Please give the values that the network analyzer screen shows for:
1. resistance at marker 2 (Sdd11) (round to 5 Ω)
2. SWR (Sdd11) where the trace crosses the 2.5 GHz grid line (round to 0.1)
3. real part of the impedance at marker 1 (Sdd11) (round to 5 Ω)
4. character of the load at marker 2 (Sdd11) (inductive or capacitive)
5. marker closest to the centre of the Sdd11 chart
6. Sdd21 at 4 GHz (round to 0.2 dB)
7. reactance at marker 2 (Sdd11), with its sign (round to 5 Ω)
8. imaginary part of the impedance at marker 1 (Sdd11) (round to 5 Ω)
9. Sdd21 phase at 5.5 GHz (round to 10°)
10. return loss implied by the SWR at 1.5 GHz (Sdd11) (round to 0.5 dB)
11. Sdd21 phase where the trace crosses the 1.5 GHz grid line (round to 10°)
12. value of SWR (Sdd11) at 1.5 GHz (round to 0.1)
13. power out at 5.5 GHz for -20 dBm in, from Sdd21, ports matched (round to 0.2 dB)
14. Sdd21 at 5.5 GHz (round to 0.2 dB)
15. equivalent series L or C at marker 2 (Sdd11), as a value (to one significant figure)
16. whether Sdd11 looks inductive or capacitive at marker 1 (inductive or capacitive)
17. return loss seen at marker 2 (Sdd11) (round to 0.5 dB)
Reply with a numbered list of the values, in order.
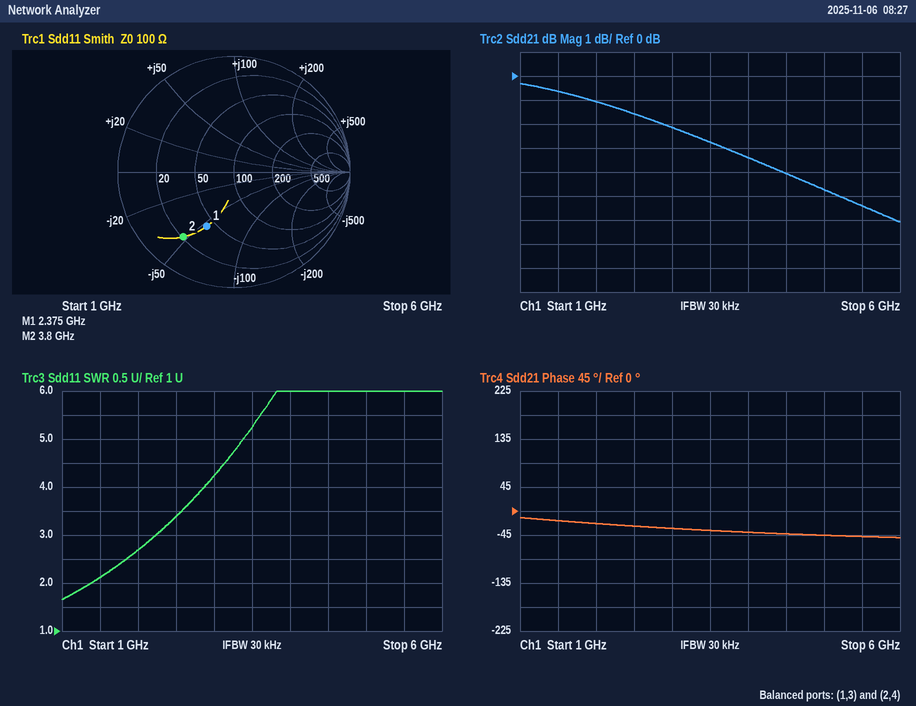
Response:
1. 20 Ω
2. 3.4
3. 40 Ω
4. capacitive
5. marker 1
6. -3.4 dB
7. -45 Ω
8. -55 Ω
9. -50°
10. 9.0 dB
11. -20°
12. 2.1
13. -25.4 dBm
14. -5.4 dB
15. 900 fF
16. capacitive
17. 3.0 dB
